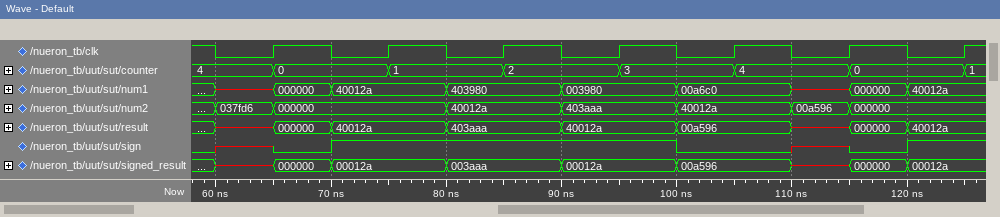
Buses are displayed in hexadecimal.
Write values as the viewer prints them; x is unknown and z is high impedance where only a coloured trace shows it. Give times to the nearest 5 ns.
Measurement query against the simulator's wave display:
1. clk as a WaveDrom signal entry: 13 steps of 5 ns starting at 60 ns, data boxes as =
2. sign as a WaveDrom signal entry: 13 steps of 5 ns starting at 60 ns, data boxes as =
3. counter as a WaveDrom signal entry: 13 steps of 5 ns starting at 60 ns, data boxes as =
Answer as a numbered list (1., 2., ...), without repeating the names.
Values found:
1. {name: 'clk', wave: '0101010101010'}
2. {name: 'sign', wave: 'x01.....0.x01'}
3. {name: 'counter', wave: '==.=.=.=.=.=.', data: '4 0 1 2 3 4 0'}
